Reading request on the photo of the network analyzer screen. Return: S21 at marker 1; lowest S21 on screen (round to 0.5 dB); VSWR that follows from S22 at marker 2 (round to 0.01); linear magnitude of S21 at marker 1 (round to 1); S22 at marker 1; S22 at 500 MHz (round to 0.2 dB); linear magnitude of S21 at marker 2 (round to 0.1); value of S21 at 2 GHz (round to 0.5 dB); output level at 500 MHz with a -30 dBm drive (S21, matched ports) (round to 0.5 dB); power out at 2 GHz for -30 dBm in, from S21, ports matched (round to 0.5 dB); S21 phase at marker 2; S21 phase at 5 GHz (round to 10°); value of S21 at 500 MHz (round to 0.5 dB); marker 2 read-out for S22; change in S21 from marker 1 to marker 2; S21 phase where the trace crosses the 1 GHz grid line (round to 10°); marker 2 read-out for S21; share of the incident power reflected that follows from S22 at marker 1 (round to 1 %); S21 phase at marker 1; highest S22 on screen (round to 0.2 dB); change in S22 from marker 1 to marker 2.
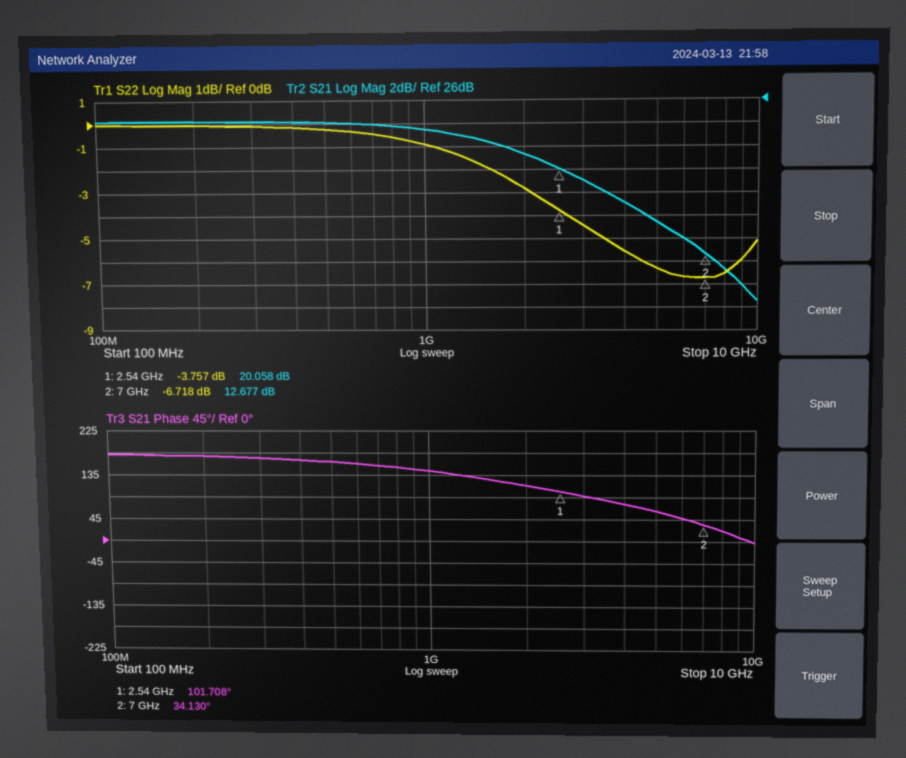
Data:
20.058 dB
8.5 dB
2.71
10
-3.757 dB
-0.2 dB
4.3
21.5 dB
-6.0 dBm
-8.5 dBm
34.130°
60°
24.0 dB
-6.718 dB
-7.381 dB
140°
12.677 dB
42 %
101.708°
0.0 dB
-2.961 dB
